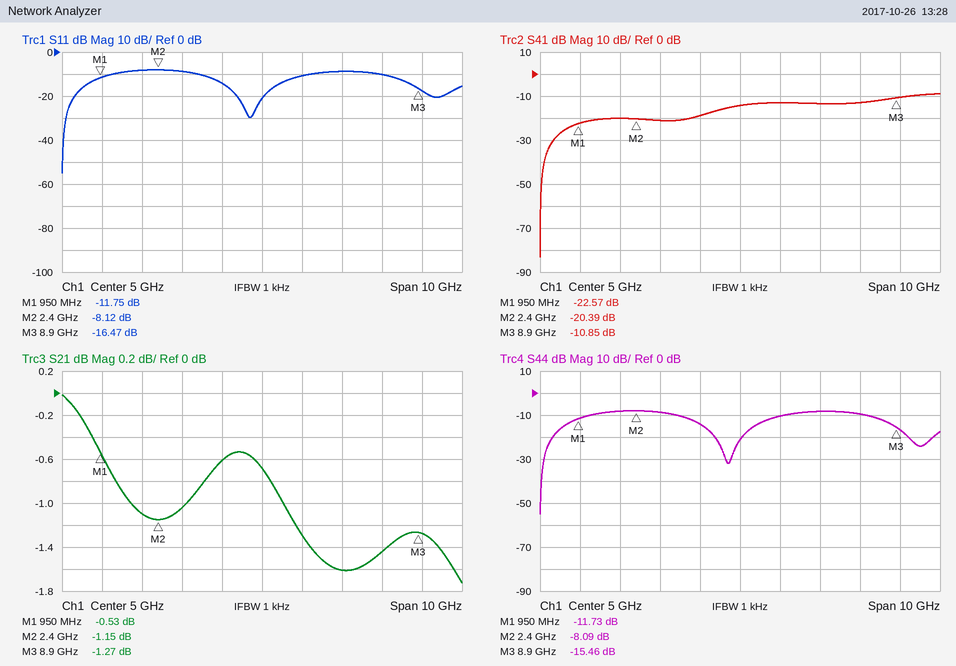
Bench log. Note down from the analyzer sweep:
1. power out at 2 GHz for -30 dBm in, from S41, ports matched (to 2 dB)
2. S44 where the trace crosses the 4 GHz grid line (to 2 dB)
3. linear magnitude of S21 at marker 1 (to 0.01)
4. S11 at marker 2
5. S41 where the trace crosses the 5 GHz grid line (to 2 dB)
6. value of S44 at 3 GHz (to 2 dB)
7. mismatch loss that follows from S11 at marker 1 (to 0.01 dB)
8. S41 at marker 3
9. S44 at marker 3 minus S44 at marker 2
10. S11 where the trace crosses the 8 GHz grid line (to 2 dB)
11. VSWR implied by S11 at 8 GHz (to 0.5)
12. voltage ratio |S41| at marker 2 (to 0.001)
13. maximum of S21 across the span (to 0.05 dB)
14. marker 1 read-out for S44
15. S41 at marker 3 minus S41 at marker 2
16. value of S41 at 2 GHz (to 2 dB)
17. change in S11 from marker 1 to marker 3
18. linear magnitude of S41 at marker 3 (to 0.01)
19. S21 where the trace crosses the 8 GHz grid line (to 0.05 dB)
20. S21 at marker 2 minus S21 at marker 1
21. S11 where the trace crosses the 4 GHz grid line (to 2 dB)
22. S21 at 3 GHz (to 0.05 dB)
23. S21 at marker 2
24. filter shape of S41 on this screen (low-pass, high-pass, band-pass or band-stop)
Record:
-50 dBm
-14 dB
0.94
-8.12 dB
-14 dB
-8 dB
0.30 dB
-10.85 dB
-7.37 dB
-10 dB
2.0
0.096
0.00 dB
-11.73 dB
9.54 dB
-20 dB
-4.72 dB
0.29
-1.45 dB
-0.62 dB
-14 dB
-1.05 dB
-1.15 dB
high-pass
